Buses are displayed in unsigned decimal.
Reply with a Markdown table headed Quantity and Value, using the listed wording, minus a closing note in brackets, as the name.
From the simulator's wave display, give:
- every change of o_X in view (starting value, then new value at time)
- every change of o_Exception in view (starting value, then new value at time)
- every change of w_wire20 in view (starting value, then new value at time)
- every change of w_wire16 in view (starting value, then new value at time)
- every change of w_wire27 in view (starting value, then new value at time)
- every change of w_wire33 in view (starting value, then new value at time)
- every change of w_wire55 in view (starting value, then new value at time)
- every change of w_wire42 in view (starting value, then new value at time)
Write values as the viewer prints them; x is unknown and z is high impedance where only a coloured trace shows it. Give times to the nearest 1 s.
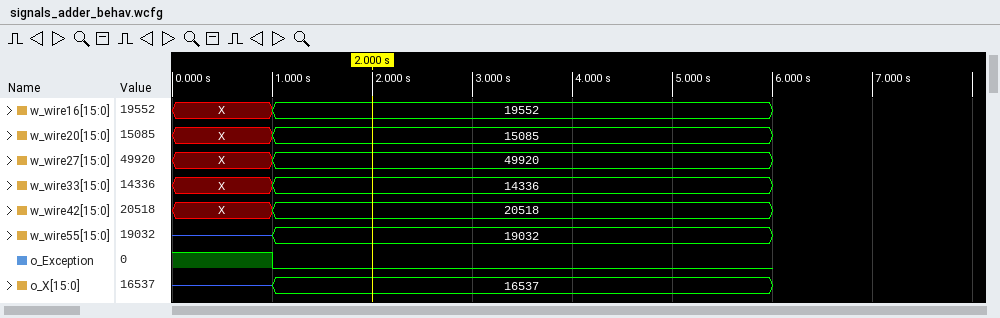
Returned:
| Quantity | Value |
|---|---|
| every change of o_X in view | z, 16537 at 1 s |
| every change of o_Exception in view | 1, 0 at 1 s |
| every change of w_wire20 in view | X, 15085 at 1 s |
| every change of w_wire16 in view | X, 19552 at 1 s |
| every change of w_wire27 in view | X, 49920 at 1 s |
| every change of w_wire33 in view | X, 14336 at 1 s |
| every change of w_wire55 in view | z, 19032 at 1 s |
| every change of w_wire42 in view | X, 20518 at 1 s |
